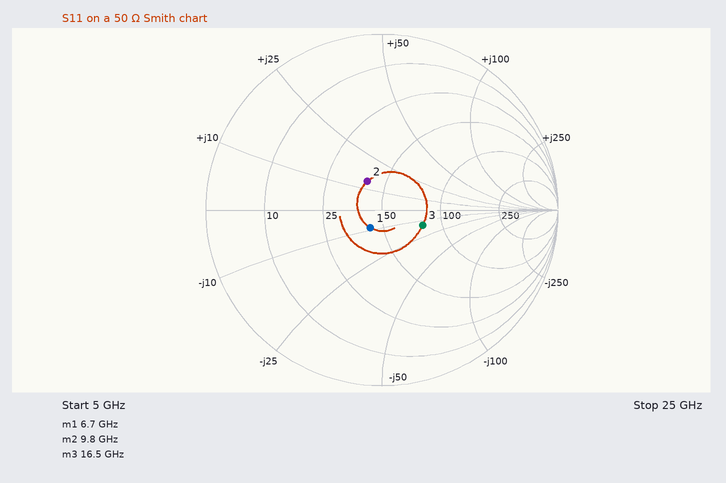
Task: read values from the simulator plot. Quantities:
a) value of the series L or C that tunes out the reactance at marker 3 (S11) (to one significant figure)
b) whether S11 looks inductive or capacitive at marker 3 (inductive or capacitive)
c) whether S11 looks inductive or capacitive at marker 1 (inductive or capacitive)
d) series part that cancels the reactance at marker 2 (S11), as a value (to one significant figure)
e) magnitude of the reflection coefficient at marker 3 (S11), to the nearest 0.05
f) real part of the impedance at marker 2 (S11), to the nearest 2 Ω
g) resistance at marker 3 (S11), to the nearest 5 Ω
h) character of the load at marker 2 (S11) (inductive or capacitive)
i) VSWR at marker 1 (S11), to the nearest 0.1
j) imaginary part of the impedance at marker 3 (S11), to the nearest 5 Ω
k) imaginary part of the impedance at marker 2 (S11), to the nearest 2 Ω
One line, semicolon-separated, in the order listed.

100 pH; capacitive; capacitive; 1 pF; 0.25; 40 Ω; 80 Ω; inductive; 1.3; -15 Ω; +14 Ω
